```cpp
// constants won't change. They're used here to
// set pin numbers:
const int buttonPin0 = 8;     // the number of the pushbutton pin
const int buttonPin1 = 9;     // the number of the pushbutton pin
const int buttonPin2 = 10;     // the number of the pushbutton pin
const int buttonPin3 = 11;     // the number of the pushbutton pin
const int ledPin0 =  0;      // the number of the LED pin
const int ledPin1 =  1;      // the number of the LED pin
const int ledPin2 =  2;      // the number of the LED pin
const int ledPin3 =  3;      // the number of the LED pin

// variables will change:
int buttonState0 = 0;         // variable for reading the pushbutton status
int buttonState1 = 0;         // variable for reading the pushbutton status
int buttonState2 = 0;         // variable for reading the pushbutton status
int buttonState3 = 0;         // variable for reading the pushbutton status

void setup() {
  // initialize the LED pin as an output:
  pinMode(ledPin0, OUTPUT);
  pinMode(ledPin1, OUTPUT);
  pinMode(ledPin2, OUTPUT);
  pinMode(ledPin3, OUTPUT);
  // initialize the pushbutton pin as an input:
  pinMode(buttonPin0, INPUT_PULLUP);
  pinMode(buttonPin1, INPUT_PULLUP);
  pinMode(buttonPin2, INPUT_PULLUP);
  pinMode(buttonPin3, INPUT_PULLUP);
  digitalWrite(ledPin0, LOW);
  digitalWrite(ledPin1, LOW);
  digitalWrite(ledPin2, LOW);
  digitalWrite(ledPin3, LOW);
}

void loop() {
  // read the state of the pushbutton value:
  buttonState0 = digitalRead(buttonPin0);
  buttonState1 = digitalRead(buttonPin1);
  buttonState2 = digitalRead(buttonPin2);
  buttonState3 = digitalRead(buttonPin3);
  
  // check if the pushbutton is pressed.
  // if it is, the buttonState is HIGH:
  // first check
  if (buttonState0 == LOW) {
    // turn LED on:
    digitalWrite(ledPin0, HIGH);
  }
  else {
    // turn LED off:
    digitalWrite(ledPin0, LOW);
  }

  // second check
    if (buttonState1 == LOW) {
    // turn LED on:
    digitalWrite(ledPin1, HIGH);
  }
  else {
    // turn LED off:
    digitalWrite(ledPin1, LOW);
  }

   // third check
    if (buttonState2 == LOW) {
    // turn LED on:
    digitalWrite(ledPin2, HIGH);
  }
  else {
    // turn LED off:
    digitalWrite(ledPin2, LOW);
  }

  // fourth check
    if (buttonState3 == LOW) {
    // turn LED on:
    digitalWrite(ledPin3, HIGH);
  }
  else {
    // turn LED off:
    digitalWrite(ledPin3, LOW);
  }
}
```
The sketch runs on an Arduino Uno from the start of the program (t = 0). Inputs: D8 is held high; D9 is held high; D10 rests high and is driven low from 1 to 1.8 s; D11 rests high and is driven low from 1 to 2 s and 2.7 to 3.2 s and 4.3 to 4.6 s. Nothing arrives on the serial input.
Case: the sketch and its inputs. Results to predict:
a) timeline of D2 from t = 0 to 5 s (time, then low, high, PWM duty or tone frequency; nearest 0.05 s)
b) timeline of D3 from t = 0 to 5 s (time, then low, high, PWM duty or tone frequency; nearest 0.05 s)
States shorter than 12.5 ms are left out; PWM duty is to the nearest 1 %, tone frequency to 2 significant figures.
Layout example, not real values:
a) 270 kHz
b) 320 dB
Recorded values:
a) 0 s low; 1 s high; 1.8 s low
b) 0 s low; 1 s high; 2 s low; 2.7 s high; 3.2 s low; 4.3 s high; 4.6 s low
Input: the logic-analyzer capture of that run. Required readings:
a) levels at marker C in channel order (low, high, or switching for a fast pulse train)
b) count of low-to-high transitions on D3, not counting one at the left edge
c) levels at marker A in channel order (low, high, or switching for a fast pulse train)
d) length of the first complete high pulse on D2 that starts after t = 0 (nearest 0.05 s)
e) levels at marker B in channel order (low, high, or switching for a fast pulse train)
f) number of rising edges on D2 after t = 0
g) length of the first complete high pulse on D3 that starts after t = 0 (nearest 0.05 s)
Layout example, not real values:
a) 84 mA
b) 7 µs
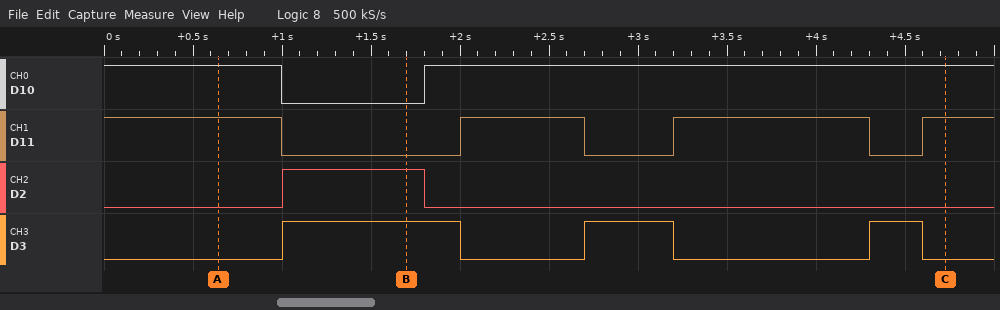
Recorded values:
a) D10 high, D11 high, D2 low, D3 low
b) 3
c) D10 high, D11 high, D2 low, D3 low
d) 0.80 s
e) D10 low, D11 low, D2 high, D3 high
f) 1
g) 1.00 s
